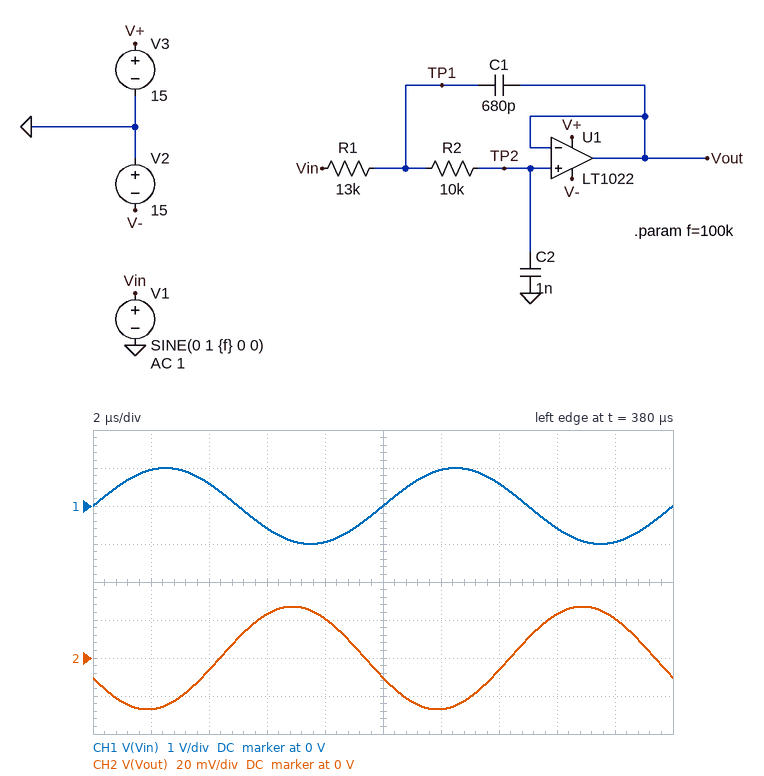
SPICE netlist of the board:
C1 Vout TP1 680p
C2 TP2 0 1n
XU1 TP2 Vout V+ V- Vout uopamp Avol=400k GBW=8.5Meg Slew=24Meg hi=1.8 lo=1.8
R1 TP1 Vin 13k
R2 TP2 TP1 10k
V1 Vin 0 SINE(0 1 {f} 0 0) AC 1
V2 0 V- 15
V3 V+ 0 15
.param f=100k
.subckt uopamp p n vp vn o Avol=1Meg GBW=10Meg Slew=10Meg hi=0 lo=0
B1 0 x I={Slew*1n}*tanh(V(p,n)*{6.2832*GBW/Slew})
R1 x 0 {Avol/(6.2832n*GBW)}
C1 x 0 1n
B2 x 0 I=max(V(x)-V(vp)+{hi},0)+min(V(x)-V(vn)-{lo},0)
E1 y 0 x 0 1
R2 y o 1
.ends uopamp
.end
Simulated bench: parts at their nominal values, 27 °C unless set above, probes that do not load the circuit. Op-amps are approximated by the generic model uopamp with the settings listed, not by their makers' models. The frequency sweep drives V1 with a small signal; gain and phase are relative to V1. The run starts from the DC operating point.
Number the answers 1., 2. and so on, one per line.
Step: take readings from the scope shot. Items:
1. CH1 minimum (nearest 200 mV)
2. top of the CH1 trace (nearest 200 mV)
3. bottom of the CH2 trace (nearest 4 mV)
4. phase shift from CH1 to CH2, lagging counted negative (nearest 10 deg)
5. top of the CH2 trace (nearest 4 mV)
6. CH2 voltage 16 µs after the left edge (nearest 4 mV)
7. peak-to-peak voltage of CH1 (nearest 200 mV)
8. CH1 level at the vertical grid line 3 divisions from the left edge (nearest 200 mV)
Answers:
1. -1.0 V
2. 1.0 V
3. -28 mV
4. -160 deg
5. 28 mV
6. 24 mV
7. 2.0 V
8. -600 mV
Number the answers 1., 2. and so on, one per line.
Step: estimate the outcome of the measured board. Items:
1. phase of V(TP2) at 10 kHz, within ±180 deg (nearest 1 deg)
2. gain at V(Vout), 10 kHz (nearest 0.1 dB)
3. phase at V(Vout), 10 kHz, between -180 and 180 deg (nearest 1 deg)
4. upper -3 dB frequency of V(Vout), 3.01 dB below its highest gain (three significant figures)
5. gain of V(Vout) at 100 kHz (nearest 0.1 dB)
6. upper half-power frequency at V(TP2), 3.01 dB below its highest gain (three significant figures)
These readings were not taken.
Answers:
1. -66 deg
2. -4.0 dB
3. -66 deg
4. 8.24 kHz
5. -31.3 dB
6. 8.24 kHz
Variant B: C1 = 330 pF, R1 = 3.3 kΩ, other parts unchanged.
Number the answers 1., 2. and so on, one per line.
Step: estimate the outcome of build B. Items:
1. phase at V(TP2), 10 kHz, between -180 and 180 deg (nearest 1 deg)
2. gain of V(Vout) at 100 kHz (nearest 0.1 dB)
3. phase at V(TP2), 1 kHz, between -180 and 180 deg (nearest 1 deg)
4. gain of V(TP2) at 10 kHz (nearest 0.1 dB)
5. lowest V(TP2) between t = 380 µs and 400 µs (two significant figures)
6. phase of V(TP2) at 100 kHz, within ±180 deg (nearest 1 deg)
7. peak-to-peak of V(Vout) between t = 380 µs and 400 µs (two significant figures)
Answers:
1. -41 deg
2. -19.1 dB
3. -5 deg
4. -2.1 dB
5. -110 mV
6. -112 deg
7. 220 mV
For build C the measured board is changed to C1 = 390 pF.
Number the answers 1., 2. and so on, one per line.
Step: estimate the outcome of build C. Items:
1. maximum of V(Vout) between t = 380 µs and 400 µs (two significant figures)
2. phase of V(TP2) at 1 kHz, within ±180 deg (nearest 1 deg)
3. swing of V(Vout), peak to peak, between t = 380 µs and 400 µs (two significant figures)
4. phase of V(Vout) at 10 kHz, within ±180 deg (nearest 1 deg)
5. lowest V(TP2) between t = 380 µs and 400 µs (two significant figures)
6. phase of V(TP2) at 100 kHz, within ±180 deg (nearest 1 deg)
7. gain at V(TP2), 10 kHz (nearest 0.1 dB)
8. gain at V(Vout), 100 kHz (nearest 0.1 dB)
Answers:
1. 42 mV
2. -8 deg
3. 84 mV
4. -61 deg
5. -42 mV
6. -143 deg
7. -4.4 dB
8. -27.6 dB
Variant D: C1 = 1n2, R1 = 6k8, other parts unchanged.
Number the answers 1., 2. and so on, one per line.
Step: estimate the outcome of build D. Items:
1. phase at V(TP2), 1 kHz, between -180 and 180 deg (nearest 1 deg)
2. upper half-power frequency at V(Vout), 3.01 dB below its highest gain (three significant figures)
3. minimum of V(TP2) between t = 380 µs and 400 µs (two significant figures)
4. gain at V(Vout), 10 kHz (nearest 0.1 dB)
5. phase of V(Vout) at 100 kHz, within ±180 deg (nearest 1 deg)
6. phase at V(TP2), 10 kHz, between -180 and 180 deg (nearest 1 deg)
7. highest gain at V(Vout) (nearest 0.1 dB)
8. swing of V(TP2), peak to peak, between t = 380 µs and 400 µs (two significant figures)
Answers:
1. -6 deg
2. 12.6 kHz
3. -30 mV
4. -2.0 dB
5. -162 deg
6. -57 deg
7. 0 dB
8. 61 mV
